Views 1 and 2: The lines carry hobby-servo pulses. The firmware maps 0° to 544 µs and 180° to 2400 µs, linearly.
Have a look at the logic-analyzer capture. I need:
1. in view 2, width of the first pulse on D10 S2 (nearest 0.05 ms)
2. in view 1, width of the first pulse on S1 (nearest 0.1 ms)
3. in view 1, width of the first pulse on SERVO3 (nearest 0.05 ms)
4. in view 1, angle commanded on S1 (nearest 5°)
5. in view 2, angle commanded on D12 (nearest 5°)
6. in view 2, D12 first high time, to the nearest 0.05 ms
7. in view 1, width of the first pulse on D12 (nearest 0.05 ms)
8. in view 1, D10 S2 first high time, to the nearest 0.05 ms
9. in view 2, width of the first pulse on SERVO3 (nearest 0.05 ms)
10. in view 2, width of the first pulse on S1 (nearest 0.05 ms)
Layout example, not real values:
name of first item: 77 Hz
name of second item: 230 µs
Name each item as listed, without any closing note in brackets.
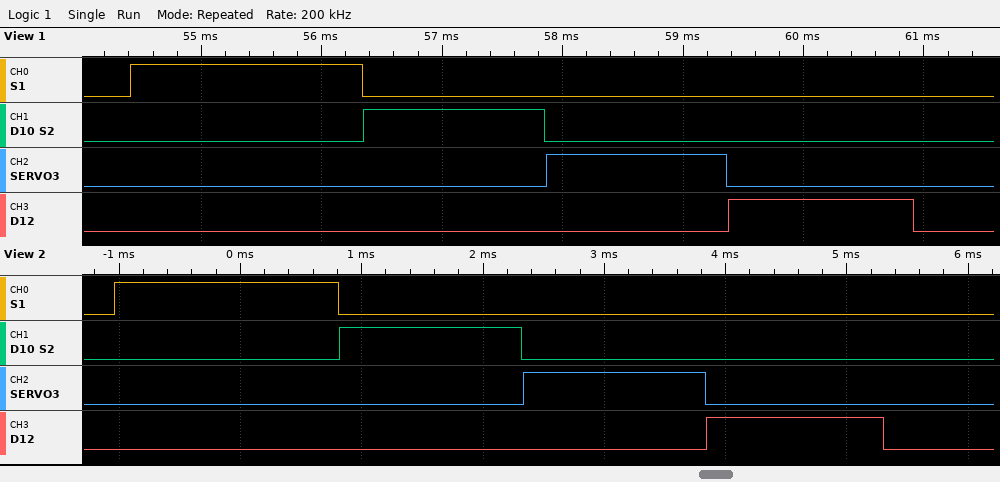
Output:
in view 2, width of the first pulse on D10 S2: 1.50 ms
in view 1, width of the first pulse on S1: 1.9 ms
in view 1, width of the first pulse on SERVO3: 1.50 ms
in view 1, angle commanded on S1: 135°
in view 2, angle commanded on D12: 90°
in view 2, D12 first high time, to the nearest 0.05 ms: 1.45 ms
in view 1, width of the first pulse on D12: 1.55 ms
in view 1, D10 S2 first high time, to the nearest 0.05 ms: 1.50 ms
in view 2, width of the first pulse on SERVO3: 1.50 ms
in view 2, width of the first pulse on S1: 1.85 ms
